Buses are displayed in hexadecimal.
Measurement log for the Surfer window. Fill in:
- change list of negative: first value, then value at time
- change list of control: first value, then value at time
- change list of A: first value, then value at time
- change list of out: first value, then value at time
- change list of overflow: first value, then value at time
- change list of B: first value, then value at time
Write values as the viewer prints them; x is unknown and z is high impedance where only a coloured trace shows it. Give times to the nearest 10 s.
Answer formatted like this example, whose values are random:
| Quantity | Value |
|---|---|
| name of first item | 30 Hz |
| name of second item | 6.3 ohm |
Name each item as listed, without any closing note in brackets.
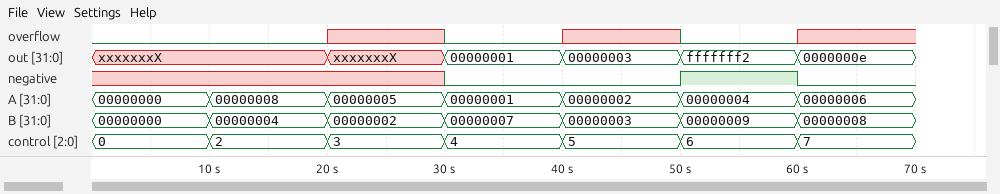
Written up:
| Quantity | Value |
|---|---|
| change list of negative: first value, then value at time | x, 0 at 30 s, 1 at 50 s, 0 at 60 s |
| change list of control: first value, then value at time | 0, 2 at 10 s, 3 at 20 s, 4 at 30 s, 5 at 40 s, 6 at 50 s, 7 at 60 s |
| change list of A: first value, then value at time | 00000000, 00000008 at 10 s, 00000005 at 20 s, 00000001 at 30 s, 00000002 at 40 s, 00000004 at 50 s, 00000006 at 60 s |
| change list of out: first value, then value at time | xxxxxxxX, xxxxxxxX at 20 s, 00000001 at 30 s, 00000003 at 40 s, fffffff2 at 50 s, 0000000e at 60 s |
| change list of overflow: first value, then value at time | 0, x at 20 s, 0 at 30 s, x at 40 s, 0 at 50 s, x at 60 s |
| change list of B: first value, then value at time | 00000000, 00000004 at 10 s, 00000002 at 20 s, 00000007 at 30 s, 00000003 at 40 s, 00000009 at 50 s, 00000008 at 60 s |
